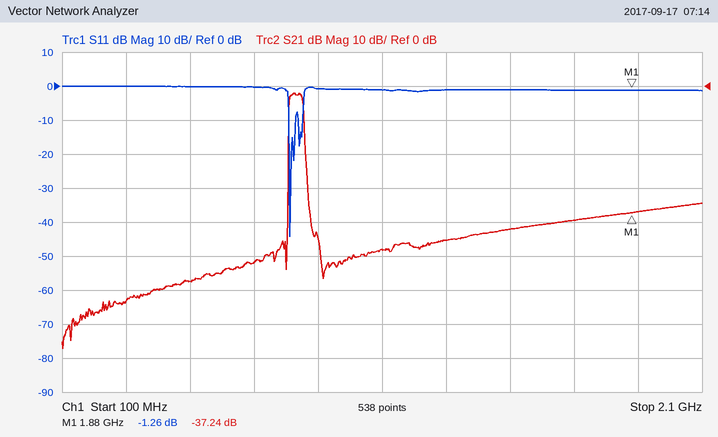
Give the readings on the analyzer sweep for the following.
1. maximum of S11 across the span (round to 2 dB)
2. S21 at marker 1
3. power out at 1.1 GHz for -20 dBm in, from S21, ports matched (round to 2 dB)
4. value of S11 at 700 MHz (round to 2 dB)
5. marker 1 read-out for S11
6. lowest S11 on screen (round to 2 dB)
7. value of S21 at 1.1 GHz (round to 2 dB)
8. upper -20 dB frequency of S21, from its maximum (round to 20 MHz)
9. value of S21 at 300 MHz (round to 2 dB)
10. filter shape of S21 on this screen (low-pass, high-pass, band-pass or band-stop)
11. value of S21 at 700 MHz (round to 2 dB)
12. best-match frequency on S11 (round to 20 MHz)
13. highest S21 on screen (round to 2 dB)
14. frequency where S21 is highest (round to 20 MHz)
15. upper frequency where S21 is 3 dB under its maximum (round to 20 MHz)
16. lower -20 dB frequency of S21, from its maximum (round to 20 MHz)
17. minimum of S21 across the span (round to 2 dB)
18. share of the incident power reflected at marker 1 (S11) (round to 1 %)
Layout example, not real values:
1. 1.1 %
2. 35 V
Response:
1. 0 dB
2. -37.24 dB
3. -68 dBm
4. 0 dB
5. -1.26 dB
6. -44 dB
7. -48 dB
8. 860 MHz
9. -64 dB
10. band-pass
11. -52 dB
12. 820 MHz
13. -2 dB
14. 820 MHz
15. 860 MHz
16. 800 MHz
17. -78 dB
18. 75 %
